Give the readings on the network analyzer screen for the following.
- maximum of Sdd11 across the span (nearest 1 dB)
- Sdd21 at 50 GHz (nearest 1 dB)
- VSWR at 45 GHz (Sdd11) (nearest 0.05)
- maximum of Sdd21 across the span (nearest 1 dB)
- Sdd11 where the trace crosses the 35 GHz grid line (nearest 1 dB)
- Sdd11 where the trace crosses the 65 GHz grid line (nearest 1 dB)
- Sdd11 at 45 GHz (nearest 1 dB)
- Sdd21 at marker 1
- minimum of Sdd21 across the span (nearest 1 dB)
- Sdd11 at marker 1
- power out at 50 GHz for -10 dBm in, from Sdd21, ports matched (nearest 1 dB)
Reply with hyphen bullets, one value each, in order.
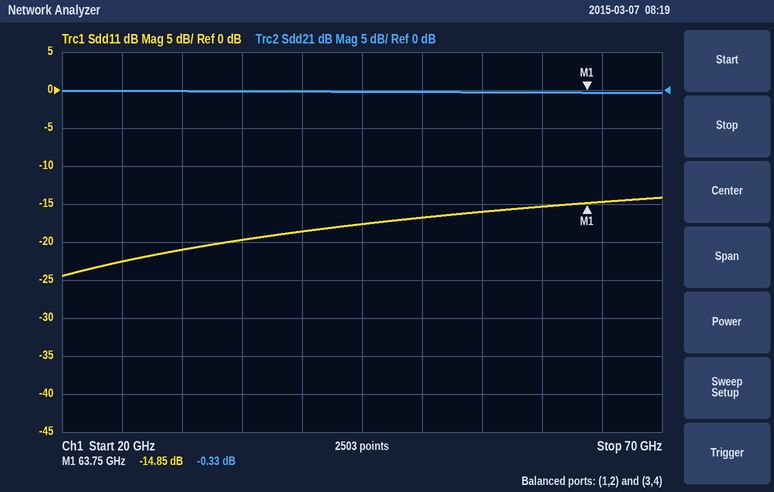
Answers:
- -14 dB
- 0 dB
- 1.30
- 0 dB
- -20 dB
- -15 dB
- -18 dB
- -0.33 dB
- 0 dB
- -14.85 dB
- -10 dBm
